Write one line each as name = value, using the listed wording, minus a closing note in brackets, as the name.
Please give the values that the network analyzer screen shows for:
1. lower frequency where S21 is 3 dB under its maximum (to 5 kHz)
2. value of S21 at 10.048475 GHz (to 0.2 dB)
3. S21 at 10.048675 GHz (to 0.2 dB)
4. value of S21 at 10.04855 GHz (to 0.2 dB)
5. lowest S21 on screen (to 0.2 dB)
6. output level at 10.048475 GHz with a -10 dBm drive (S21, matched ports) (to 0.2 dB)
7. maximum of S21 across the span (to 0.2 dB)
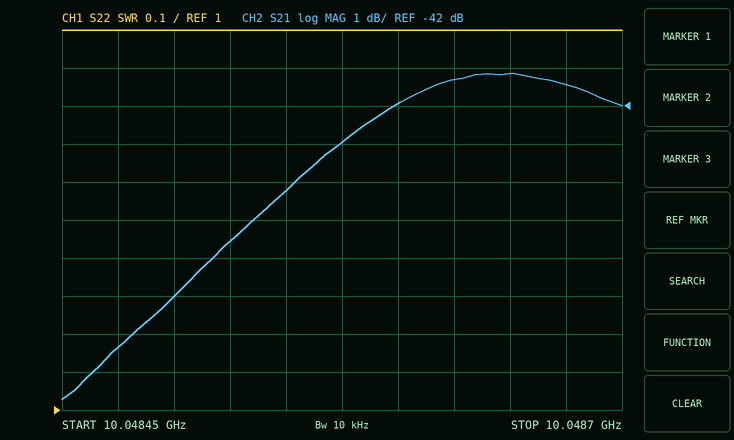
lower frequency where S21 is 3 dB under its maximum = 10.048550 GHz
value of S21 at 10.048475 GHz = -48.4 dB
S21 at 10.048675 GHz = -41.4 dB
value of S21 at 10.04855 GHz = -44.2 dB
lowest S21 on screen = -49.8 dB
output level at 10.048475 GHz with a -10 dBm drive (S21, matched ports) = -58.4 dBm
maximum of S21 across the span = -41.2 dB
